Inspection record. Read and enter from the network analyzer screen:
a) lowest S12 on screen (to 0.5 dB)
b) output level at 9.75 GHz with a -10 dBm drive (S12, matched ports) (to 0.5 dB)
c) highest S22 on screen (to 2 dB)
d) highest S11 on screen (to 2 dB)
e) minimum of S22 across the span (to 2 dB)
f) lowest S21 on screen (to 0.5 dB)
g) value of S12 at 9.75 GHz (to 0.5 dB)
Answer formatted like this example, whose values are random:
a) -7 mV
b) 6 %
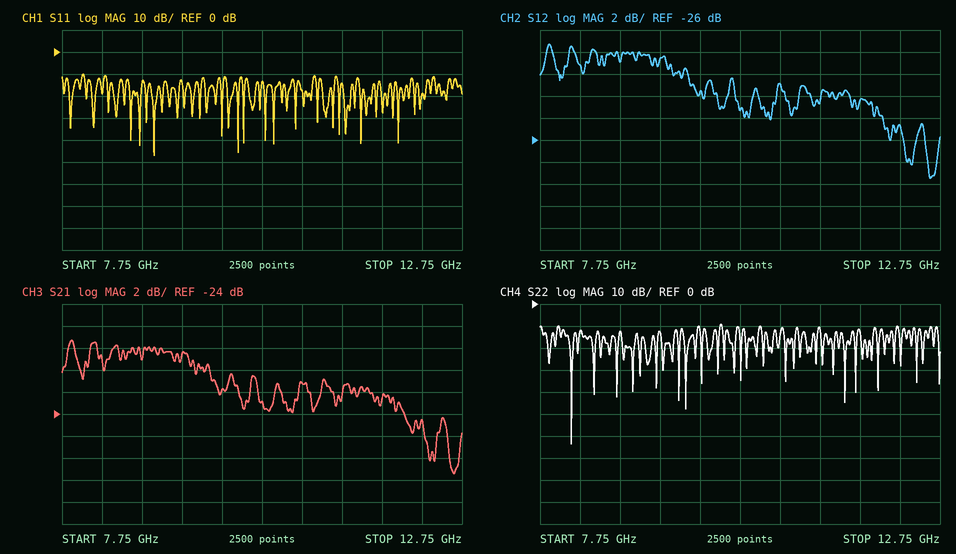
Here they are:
a) -29.5 dB
b) -31.5 dBm
c) -10 dB
d) -10 dB
e) -64 dB
f) -29.5 dB
g) -21.5 dB
